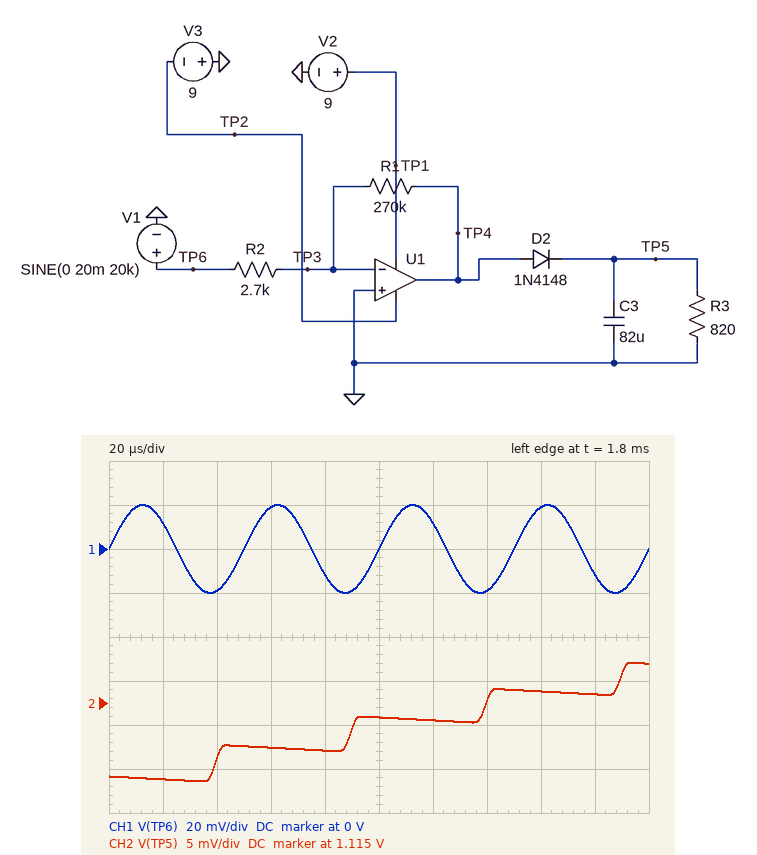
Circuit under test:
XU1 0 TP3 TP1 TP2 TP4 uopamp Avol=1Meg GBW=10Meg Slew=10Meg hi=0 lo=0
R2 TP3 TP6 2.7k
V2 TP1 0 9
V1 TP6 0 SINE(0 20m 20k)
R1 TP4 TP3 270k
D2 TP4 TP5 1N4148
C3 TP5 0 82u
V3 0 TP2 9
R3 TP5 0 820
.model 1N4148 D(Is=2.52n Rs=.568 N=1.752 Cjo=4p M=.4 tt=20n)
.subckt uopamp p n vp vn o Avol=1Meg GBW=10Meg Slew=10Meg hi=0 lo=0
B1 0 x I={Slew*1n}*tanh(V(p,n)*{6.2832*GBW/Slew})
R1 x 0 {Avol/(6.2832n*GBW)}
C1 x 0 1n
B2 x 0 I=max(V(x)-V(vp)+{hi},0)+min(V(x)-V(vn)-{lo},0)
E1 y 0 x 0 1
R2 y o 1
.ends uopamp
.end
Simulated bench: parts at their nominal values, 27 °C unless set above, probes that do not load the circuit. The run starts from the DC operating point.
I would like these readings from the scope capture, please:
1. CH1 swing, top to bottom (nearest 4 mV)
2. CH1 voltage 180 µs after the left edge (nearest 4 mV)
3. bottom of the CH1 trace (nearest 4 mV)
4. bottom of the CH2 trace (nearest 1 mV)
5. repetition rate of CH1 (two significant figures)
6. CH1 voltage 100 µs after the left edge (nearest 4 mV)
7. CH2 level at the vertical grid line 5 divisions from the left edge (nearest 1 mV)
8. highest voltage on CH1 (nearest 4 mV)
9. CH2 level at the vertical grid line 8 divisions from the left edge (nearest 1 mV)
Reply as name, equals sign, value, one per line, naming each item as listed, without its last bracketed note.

CH1 swing, top to bottom = 40 mV
CH1 voltage 180 µs after the left edge = -12 mV
bottom of the CH1 trace = -20 mV
bottom of the CH2 trace = 1.106 V
repetition rate of CH1 = 20 kHz
CH1 voltage 100 µs after the left edge = 0 V
CH2 level at the vertical grid line 5 divisions from the left edge = 1.113 V
highest voltage on CH1 = 20 mV
CH2 level at the vertical grid line 8 divisions from the left edge = 1.116 V
